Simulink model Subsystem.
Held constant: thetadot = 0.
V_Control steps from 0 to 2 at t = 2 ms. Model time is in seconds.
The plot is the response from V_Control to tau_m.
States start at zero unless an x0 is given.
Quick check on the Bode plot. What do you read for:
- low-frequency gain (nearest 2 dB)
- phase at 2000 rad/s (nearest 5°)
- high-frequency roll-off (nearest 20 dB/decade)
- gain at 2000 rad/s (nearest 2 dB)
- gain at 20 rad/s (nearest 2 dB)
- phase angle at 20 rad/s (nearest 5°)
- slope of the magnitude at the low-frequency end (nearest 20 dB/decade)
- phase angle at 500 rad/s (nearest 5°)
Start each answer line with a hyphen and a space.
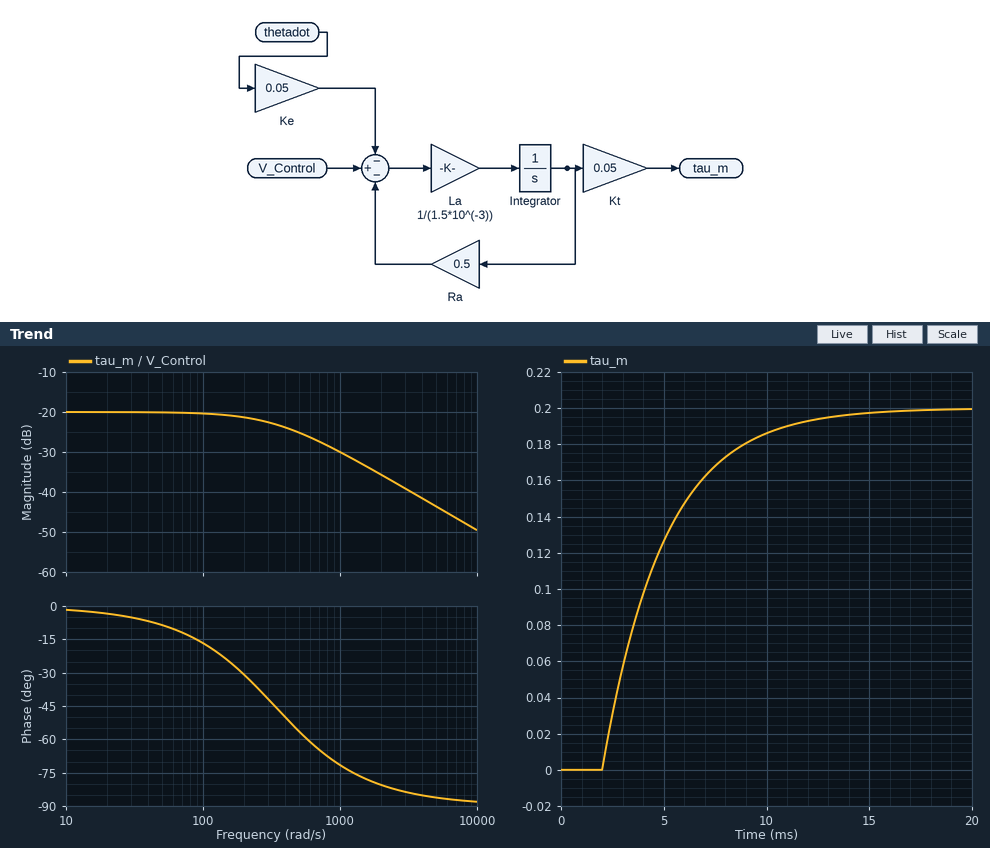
- -20 dB
- -80°
- -20 dB/decade
- -36 dB
- -20 dB
- -5°
- 0 dB/decade
- -55°
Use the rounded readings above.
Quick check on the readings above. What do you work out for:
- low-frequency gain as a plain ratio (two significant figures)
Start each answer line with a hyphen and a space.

- 0.10
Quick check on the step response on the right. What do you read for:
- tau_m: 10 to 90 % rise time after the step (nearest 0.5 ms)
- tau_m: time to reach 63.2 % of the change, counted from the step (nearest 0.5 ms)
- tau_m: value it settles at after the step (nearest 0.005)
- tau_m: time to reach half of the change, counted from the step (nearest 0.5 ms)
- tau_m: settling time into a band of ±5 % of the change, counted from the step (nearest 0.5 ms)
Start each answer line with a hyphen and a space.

- 6.5 ms
- 3.0 ms
- 0.200
- 2.0 ms
- 9.0 ms
